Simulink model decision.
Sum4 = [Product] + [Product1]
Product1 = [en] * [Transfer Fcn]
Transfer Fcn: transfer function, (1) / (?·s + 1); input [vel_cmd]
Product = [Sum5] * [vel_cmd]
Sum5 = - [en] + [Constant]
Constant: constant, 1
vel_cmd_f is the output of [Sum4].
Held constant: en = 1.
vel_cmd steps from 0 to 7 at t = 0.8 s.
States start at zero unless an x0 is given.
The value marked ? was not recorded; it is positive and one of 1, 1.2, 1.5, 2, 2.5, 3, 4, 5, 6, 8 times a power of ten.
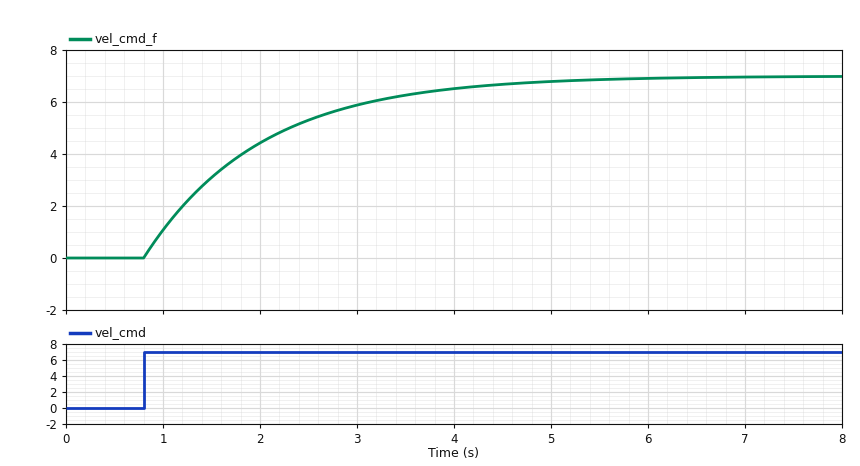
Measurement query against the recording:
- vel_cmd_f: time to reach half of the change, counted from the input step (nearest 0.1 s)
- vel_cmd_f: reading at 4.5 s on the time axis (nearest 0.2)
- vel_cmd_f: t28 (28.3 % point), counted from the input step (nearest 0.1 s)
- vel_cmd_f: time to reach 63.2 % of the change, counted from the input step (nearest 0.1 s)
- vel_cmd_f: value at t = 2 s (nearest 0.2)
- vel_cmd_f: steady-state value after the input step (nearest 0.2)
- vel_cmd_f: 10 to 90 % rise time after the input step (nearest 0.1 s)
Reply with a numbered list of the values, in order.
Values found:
1. 0.8 s
2. 6.6
3. 0.4 s
4. 1.2 s
5. 4.4
6. 7.0
7. 2.6 s
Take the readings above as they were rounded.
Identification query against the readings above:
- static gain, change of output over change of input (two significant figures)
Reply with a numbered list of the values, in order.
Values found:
1. 1.0
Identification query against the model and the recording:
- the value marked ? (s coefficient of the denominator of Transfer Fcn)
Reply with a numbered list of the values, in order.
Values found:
1. 1.2
